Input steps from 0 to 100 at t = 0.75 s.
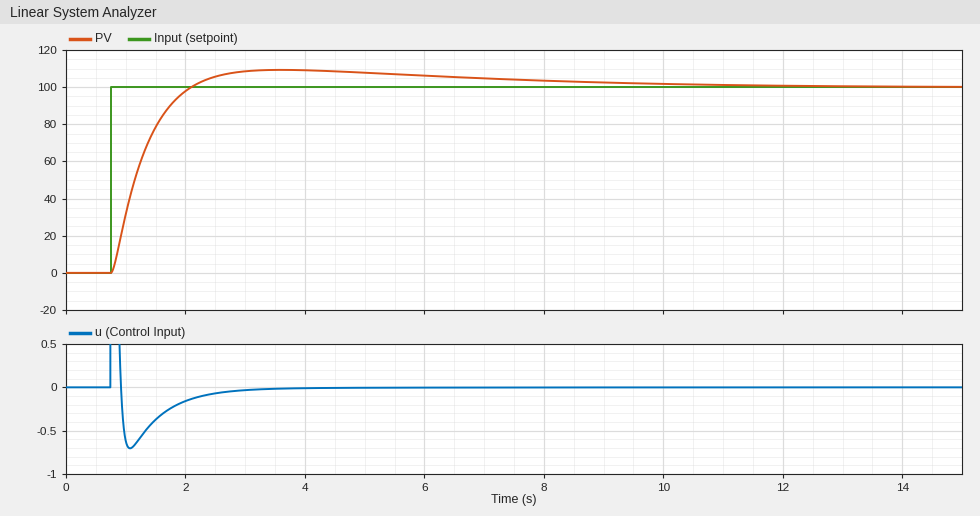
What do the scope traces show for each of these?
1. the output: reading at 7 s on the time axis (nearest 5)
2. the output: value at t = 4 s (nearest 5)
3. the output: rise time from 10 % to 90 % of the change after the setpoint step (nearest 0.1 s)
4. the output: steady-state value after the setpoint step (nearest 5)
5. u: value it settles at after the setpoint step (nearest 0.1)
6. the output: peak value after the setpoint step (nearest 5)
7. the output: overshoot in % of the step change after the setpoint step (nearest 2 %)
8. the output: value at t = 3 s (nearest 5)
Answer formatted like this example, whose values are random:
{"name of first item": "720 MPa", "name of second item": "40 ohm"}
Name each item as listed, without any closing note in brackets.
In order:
{"the output: reading at 7 s on the time axis": "105", "the output: value at t = 4 s": "110", "the output: rise time from 10 % to 90 % of the change after the setpoint step": "0.9 s", "the output: steady-state value after the setpoint step": "100", "u: value it settles at after the setpoint step": "0.0", "the output: peak value after the setpoint step": "110", "the output: overshoot in % of the step change after the setpoint step": "10 %", "the output: value at t = 3 s": "110"}
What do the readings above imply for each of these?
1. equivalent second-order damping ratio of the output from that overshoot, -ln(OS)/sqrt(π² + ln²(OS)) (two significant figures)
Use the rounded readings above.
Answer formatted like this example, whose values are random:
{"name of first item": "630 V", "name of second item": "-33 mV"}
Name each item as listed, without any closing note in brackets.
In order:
{"equivalent second-order damping ratio of the output from that overshoot, -ln(OS)/sqrt(π² + ln²(OS))": "0.59"}
